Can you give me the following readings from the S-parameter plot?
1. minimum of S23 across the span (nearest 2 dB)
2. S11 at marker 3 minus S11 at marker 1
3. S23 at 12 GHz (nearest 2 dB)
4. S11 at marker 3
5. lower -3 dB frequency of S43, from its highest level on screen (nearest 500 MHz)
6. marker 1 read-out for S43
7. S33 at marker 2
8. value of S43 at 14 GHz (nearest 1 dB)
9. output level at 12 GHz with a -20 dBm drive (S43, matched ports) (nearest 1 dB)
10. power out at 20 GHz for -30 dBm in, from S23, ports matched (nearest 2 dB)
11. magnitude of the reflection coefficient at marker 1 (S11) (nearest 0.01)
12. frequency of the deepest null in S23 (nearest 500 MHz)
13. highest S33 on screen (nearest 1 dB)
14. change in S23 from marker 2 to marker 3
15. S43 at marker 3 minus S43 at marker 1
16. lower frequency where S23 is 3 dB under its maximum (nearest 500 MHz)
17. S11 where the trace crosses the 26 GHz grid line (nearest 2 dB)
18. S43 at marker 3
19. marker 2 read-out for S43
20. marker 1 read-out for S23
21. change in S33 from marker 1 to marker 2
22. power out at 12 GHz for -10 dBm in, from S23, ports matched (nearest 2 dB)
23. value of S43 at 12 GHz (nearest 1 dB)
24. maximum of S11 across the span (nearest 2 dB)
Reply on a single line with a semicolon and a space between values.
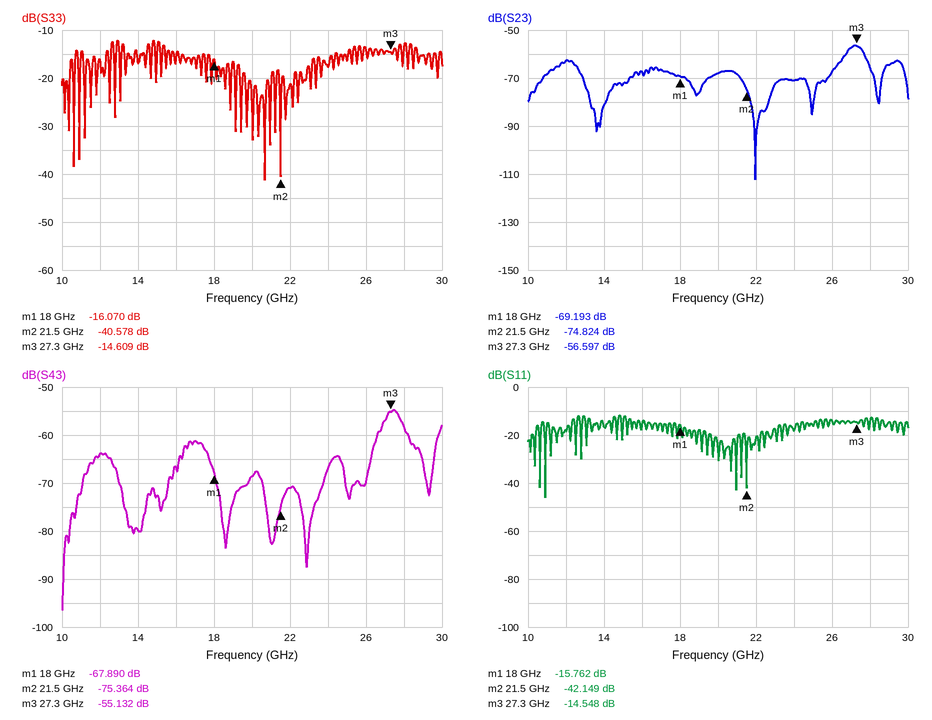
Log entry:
-112 dB; 1.214 dB; -62 dB; -14.548 dB; 27.0 GHz; -67.890 dB; -40.578 dB; -80 dB; -84 dBm; -98 dBm; 0.16; 22.0 GHz; -12 dB; 18.227 dB; 12.758 dB; 27.0 GHz; -14 dB; -55.132 dB; -75.364 dB; -69.193 dB; -24.508 dB; -72 dBm; -64 dB; -12 dB
